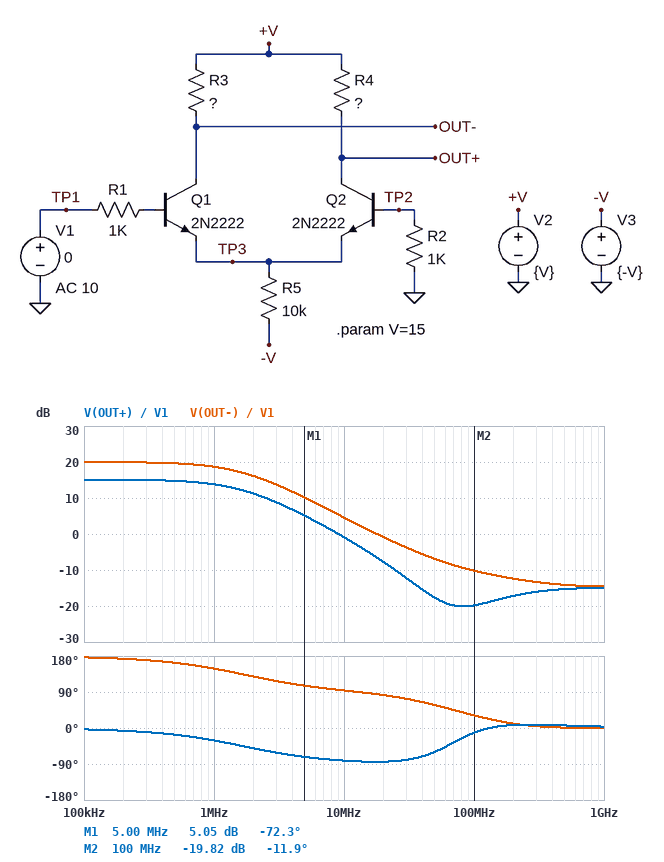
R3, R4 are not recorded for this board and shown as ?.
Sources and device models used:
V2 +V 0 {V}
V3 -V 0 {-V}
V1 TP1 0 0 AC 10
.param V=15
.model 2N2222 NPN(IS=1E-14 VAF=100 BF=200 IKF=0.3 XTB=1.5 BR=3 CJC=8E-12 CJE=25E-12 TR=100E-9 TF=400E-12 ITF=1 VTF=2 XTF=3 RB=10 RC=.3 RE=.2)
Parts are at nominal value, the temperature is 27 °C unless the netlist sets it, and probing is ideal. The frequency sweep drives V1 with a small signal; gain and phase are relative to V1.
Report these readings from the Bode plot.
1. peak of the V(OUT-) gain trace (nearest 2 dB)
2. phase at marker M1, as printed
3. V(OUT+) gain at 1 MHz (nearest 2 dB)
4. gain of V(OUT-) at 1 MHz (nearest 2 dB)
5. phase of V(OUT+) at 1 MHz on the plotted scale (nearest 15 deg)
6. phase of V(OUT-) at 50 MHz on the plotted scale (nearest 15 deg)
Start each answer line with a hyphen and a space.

- 20 dB
- -72.3 deg
- 14 dB
- 18 dB
- -30 deg
- 60 deg
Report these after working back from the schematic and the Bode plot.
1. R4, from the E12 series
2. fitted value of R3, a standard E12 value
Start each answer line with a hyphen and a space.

- 470 Ω
- 820 Ω
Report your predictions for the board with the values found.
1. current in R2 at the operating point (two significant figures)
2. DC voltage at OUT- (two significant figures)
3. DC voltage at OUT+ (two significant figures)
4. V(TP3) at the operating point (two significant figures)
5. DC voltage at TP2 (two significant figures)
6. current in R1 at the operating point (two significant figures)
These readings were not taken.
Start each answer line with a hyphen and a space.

- 3.1 µA
- 14 V
- 15 V
- -650 mV
- -3.1 mV
- 3.1 µA
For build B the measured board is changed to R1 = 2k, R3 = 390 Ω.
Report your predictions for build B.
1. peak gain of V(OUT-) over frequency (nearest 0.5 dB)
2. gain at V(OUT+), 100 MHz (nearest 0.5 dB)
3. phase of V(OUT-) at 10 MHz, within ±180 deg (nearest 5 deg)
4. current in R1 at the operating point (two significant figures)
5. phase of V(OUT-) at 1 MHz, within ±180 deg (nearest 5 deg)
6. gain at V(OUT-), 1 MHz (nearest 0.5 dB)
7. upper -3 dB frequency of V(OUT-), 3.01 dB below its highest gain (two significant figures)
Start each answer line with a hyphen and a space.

- 13.0 dB
- -25.5 dB
- 90 deg
- 3.0 µA
- 145 deg
- 11.5 dB
- 1.4 MHz
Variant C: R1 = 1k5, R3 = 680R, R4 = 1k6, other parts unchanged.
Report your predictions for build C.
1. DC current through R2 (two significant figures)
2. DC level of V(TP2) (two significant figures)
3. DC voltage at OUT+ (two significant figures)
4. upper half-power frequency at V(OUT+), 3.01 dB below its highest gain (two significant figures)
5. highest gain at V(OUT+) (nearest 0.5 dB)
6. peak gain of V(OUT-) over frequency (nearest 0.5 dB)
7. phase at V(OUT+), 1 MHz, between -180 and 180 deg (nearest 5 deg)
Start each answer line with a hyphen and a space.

- 3.2 µA
- -3.2 mV
- 14 V
- 1.0 MHz
- 25.5 dB
- 18.0 dB
- -45 deg
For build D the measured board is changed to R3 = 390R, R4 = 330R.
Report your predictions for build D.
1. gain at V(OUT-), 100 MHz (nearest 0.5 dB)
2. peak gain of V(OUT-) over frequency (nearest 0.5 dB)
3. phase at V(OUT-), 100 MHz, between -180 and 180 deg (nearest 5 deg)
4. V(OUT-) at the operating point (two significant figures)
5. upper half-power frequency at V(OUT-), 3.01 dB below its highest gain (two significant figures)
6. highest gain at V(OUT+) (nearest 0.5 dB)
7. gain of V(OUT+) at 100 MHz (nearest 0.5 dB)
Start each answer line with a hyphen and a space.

- -14.0 dB
- 13.5 dB
- 40 deg
- 15 V
- 2.2 MHz
- 12.0 dB
- -22.0 dB
